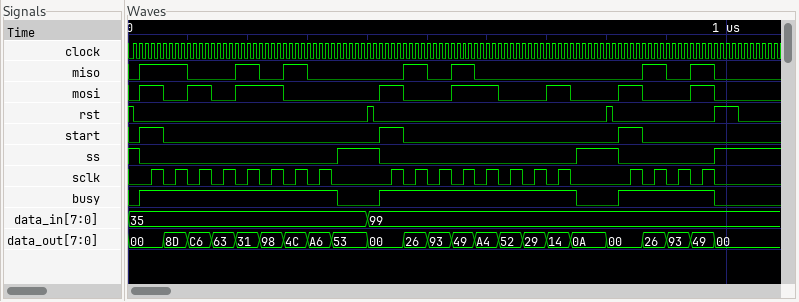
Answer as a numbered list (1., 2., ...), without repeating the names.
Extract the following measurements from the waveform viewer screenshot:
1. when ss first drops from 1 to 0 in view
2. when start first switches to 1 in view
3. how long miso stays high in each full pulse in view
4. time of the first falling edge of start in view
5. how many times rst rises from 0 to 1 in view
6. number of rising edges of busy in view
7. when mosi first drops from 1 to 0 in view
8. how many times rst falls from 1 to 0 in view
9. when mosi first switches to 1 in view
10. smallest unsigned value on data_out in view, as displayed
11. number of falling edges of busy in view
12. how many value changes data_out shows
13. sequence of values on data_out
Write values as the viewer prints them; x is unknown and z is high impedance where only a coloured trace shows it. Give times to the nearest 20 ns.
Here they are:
1. 20 ns
2. 20 ns
3. 80 ns, 40 ns, 40 ns, 40 ns, 40 ns, 40 ns, 40 ns
4. 60 ns
5. 3
6. 3
7. 60 ns
8. 4
9. 20 ns
10. 00
11. 3
12. 22
13. 00, 8D, C6, 63, 31, 98, 4C, A6, 53, 00, 26, 93, 49, A4, 52, 29, 14, 0A, 00, 26, 93, 49, 00
